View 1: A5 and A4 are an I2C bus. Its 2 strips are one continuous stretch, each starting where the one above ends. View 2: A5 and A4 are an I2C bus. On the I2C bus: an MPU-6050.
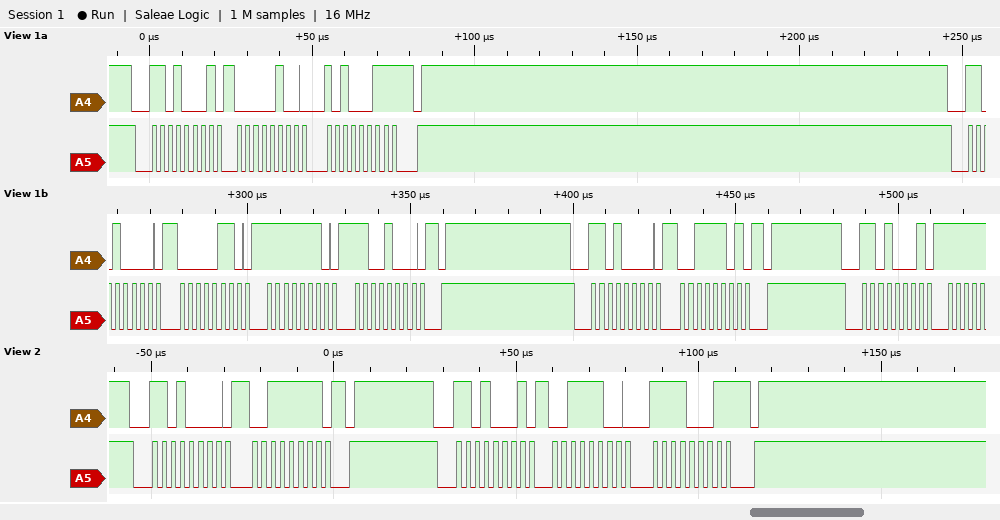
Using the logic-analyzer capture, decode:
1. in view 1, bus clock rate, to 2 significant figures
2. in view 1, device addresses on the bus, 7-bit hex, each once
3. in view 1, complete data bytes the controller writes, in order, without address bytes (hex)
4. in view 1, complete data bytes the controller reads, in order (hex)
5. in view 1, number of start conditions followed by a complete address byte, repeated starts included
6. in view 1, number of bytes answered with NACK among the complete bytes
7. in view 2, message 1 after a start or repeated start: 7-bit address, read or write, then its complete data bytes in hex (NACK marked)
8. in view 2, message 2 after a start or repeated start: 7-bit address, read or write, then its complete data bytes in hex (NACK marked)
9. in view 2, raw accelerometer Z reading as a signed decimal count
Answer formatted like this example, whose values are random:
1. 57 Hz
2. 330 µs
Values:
1. 400 kHz
2. 0x68
3. 06 FE C8 3D
4. 04 A3
5. 4
6. 1
7. 0x68 write: 3F
8. 0x68 read: 3C F1 NACK
9. 15601
